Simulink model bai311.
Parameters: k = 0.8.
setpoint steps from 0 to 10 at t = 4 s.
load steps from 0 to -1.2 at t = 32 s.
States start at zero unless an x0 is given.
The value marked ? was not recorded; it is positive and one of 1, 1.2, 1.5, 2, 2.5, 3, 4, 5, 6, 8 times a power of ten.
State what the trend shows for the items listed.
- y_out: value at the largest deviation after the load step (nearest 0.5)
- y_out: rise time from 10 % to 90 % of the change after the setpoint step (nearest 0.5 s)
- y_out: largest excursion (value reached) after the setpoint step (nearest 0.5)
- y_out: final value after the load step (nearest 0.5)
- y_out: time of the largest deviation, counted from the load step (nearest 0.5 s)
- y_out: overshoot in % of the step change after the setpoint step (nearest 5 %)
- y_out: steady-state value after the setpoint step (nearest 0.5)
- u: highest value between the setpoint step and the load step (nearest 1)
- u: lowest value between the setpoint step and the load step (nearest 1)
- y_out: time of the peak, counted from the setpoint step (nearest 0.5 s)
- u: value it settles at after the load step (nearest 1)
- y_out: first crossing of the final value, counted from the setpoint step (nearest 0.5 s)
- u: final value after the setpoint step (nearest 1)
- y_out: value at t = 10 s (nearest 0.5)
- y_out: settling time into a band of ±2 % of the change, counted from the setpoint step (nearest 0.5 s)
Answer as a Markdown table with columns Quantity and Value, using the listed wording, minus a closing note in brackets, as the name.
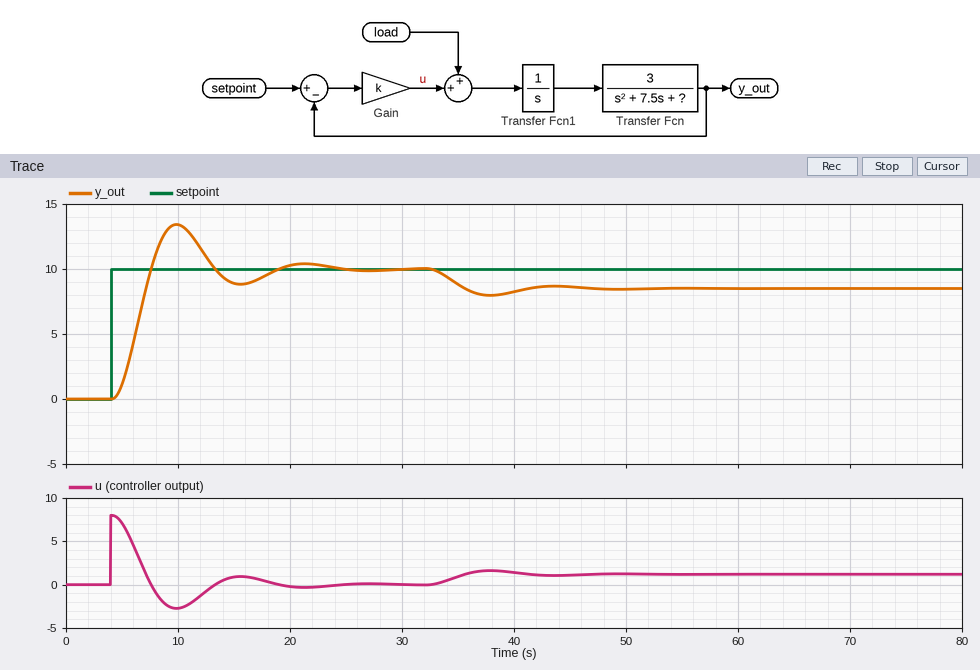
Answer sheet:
| Quantity | Value |
|---|---|
| y_out: value at the largest deviation after the load step | 8.0 |
| y_out: rise time from 10 % to 90 % of the change after the setpoint step | 2.5 s |
| y_out: largest excursion (value reached) after the setpoint step | 13.5 |
| y_out: final value after the load step | 8.5 |
| y_out: time of the largest deviation, counted from the load step | 6.0 s |
| y_out: overshoot in % of the step change after the setpoint step | 35 % |
| y_out: steady-state value after the setpoint step | 10.0 |
| u: highest value between the setpoint step and the load step | 8 |
| u: lowest value between the setpoint step and the load step | -3 |
| y_out: time of the peak, counted from the setpoint step | 6.0 s |
| u: value it settles at after the load step | 1 |
| y_out: first crossing of the final value, counted from the setpoint step | 3.5 s |
| u: final value after the setpoint step | 0 |
| y_out: value at t = 10 s | 13.5 |
| y_out: settling time into a band of ±2 % of the change, counted from the setpoint step | 19.5 s |
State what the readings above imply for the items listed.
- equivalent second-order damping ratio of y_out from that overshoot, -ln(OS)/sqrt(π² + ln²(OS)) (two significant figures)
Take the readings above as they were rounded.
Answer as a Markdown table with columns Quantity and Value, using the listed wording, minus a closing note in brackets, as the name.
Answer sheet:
| Quantity | Value |
|---|---|
| equivalent second-order damping ratio of y_out from that overshoot, -ln(OS)/sqrt(π² + ln²(OS)) | 0.32 |
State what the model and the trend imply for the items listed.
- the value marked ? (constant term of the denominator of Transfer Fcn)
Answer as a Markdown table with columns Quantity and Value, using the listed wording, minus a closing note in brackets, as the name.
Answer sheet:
| Quantity | Value |
|---|---|
| the value marked ? | 3 |
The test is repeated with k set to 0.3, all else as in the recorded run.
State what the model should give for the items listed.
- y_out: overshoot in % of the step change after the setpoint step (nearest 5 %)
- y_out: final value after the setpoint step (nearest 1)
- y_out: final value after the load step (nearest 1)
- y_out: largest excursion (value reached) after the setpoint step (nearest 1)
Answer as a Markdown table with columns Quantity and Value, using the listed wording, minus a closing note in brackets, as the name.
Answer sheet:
| Quantity | Value |
|---|---|
| y_out: overshoot in % of the step change after the setpoint step | 10 % |
| y_out: final value after the setpoint step | 10 |
| y_out: final value after the load step | 6 |
| y_out: largest excursion (value reached) after the setpoint step | 11 |
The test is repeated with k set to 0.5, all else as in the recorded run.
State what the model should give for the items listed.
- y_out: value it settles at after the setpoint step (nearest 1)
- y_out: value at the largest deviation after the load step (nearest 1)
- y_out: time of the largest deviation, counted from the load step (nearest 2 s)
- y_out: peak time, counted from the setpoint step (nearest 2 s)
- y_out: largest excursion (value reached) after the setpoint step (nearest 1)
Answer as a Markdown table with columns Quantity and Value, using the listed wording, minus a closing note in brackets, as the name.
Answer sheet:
| Quantity | Value |
|---|---|
| y_out: value it settles at after the setpoint step | 10 |
| y_out: value at the largest deviation after the load step | 7 |
| y_out: time of the largest deviation, counted from the load step | 8 s |
| y_out: peak time, counted from the setpoint step | 8 s |
| y_out: largest excursion (value reached) after the setpoint step | 12 |
